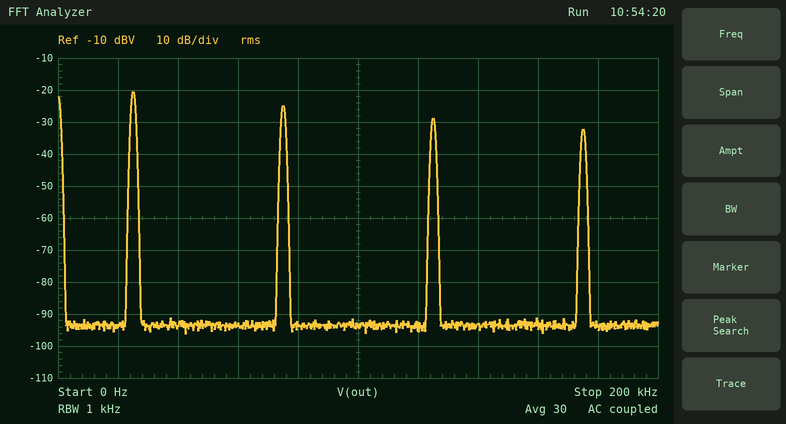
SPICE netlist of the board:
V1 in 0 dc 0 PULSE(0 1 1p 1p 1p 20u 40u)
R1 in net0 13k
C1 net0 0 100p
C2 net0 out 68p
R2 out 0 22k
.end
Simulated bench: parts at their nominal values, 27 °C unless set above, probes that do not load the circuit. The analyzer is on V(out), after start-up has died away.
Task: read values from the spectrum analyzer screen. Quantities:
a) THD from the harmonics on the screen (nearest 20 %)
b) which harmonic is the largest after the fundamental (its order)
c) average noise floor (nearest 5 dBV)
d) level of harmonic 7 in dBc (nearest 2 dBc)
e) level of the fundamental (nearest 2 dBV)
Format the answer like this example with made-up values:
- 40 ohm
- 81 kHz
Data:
- 80 %
- 3
- -95 dBV
- -12 dBc
- -20 dBV
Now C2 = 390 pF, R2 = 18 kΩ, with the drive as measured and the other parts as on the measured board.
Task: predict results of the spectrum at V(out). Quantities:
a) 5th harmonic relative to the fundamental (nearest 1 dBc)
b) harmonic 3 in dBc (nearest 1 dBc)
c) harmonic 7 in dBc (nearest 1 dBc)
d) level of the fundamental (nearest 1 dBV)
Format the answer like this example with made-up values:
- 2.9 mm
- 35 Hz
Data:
- -14 dBc
- -9 dBc
- -18 dBc
- -13 dBV
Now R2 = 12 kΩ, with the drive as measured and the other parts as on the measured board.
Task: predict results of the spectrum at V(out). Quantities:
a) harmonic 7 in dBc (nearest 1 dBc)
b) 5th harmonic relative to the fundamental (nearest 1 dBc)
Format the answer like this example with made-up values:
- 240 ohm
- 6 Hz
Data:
- -10 dBc
- -7 dBc
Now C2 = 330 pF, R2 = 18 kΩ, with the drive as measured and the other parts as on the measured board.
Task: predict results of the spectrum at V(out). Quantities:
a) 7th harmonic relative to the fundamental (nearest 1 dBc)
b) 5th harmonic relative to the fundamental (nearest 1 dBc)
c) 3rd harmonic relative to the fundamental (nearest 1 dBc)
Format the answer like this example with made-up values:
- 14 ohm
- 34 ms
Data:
- -18 dBc
- -14 dBc
- -9 dBc
